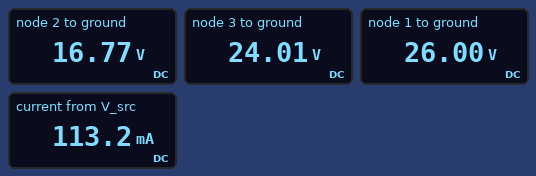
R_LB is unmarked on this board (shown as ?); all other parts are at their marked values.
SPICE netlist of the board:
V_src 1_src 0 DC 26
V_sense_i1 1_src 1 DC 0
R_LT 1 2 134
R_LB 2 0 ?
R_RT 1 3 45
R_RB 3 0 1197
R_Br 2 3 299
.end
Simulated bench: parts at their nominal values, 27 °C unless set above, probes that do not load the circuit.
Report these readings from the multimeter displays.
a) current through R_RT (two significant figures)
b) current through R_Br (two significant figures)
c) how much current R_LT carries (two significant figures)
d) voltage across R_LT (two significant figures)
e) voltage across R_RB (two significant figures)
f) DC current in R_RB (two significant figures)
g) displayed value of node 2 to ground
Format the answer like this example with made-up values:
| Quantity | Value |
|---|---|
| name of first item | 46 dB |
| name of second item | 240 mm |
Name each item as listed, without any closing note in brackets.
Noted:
| Quantity | Value |
|---|---|
| current through R_RT | 44 mA |
| current through R_Br | 24 mA |
| how much current R_LT carries | 69 mA |
| voltage across R_LT | 9.2 V |
| voltage across R_RB | 24 V |
| DC current in R_RB | 20 mA |
| displayed value of node 2 to ground | 16.77 V |
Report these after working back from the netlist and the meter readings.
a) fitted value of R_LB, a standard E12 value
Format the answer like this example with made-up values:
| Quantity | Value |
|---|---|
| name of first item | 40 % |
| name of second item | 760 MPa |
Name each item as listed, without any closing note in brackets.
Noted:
| Quantity | Value |
|---|---|
| fitted value of R_LB, a standard E12 value | 180 Ω |
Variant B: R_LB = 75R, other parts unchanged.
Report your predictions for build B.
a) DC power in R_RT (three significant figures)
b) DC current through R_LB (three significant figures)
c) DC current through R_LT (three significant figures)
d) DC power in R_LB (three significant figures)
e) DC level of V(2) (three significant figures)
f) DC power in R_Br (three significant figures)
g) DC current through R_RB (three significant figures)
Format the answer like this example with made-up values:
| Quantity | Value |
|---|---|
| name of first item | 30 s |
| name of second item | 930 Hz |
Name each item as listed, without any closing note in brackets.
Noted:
| Quantity | Value |
|---|---|
| DC power in R_RT | 161 mW |
| DC current through R_LB | 150 mA |
| DC current through R_LT | 110 mA |
| DC power in R_LB | 1.69 W |
| DC level of V(2) | 11.3 V |
| DC power in R_Br | 485 mW |
| DC current through R_RB | 19.5 mA |
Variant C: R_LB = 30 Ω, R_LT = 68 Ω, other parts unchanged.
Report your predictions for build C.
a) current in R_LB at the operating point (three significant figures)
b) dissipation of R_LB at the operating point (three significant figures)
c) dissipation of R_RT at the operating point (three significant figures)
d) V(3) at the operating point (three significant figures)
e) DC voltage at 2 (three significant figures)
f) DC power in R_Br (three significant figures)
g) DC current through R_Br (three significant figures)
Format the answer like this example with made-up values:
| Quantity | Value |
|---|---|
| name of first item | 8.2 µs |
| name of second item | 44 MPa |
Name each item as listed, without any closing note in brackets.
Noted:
| Quantity | Value |
|---|---|
| current in R_LB at the operating point | 298 mA |
| dissipation of R_LB at the operating point | 2.66 W |
| dissipation of R_RT at the operating point | 198 mW |
| V(3) at the operating point | 23.0 V |
| DC voltage at 2 | 8.94 V |
| DC power in R_Br | 663 mW |
| DC current through R_Br | 47.1 mA |
